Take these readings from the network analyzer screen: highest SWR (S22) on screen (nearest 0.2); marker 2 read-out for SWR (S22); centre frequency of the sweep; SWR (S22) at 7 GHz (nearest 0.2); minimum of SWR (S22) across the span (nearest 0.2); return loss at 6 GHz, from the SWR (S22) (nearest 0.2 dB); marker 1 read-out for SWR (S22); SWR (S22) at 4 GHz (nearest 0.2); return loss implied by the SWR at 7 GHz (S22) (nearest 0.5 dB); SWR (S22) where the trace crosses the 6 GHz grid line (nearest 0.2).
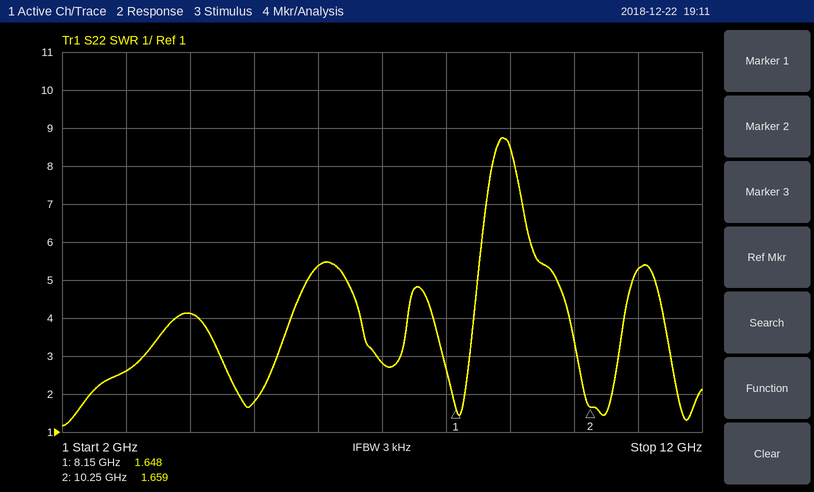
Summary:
8.8
1.659
7 GHz
2.8
1.2
3.2 dB
1.648
4.2
6.5 dB
5.4
